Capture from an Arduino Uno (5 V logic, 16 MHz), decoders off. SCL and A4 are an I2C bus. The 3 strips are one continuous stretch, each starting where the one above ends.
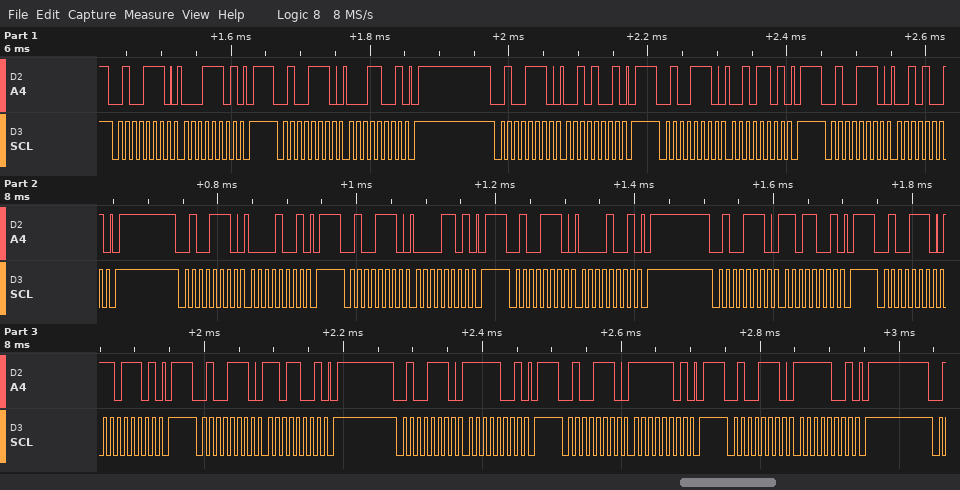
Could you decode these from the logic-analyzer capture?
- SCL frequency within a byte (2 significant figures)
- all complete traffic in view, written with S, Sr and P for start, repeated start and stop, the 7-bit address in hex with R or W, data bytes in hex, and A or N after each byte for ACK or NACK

100 kHz
S 27W A 1D A P S 27W A 19 A P S 27W A 29 A P S 27W A 2D A P S 27W A 29 A P S 27W A 09 A P S 27W A 0D A P S 27W A 09 A P S 27W A D9 A P S 27W A DD A P S 27W A D9 A P S 27W A F9 A P S 27W A FD A P S 27W A F9 A P
